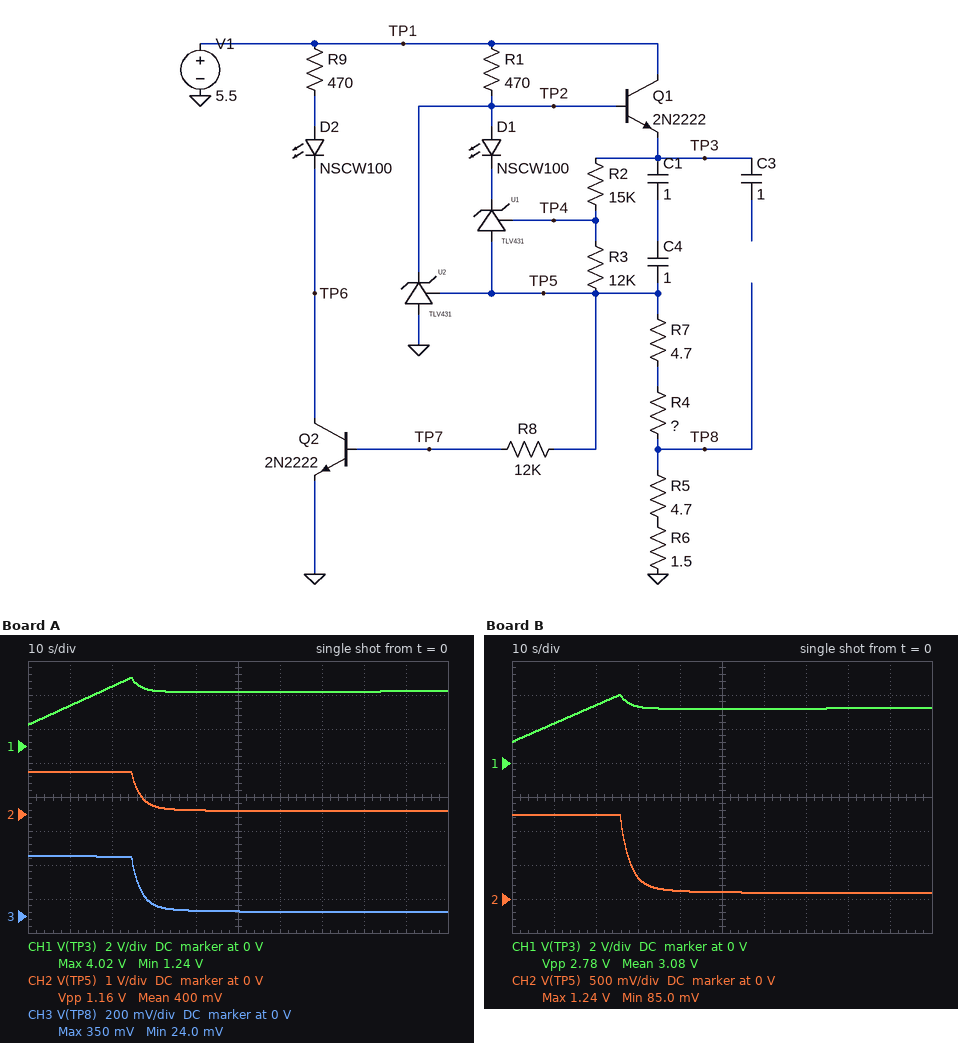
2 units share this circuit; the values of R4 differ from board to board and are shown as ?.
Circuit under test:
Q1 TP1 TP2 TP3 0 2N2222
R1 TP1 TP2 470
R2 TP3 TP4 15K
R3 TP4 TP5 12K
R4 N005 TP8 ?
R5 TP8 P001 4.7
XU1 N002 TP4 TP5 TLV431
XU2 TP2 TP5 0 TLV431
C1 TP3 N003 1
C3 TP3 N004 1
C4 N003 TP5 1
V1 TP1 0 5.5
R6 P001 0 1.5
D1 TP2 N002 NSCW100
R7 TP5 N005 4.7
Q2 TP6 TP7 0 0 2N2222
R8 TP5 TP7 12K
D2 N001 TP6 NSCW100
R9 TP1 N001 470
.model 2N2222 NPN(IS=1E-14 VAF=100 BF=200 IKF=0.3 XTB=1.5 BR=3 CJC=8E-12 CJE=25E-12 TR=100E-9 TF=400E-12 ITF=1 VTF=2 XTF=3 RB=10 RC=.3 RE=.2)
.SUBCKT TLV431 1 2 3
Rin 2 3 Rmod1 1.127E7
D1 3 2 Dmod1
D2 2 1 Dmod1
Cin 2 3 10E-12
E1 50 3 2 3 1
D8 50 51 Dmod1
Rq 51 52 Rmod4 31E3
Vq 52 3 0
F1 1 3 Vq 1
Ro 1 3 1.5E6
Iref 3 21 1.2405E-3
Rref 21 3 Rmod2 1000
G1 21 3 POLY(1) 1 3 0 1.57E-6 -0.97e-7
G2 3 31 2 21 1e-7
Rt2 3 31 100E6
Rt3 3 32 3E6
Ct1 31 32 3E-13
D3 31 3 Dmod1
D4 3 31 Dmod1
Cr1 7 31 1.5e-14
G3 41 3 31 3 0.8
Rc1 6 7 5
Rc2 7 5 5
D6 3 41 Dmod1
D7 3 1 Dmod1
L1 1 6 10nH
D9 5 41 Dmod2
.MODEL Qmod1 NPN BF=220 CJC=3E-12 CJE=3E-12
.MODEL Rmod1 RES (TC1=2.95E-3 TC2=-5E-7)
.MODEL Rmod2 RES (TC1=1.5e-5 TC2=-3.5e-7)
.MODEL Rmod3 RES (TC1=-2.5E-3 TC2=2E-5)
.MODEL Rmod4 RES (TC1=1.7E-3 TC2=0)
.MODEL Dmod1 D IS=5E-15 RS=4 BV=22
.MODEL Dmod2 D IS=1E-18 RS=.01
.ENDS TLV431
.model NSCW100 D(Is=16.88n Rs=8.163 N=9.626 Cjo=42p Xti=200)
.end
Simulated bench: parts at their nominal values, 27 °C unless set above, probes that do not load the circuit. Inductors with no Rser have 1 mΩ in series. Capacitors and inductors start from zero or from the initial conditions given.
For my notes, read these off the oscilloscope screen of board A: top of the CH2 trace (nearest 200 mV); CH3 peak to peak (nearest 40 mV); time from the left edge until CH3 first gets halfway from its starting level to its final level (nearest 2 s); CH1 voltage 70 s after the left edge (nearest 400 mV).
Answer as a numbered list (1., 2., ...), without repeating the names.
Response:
1. 1.2 V
2. 320 mV
3. 26 s
4. 3.2 V
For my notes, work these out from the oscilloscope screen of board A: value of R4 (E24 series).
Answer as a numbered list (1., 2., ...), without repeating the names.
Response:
1. 11 Ω
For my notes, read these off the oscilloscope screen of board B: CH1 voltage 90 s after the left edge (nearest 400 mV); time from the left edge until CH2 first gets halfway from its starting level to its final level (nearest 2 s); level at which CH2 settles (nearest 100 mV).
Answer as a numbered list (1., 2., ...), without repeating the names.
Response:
1. 3.2 V
2. 28 s
3. 100 mV
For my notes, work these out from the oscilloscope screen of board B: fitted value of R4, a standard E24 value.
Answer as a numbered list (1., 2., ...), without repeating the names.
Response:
1. 12 Ω
